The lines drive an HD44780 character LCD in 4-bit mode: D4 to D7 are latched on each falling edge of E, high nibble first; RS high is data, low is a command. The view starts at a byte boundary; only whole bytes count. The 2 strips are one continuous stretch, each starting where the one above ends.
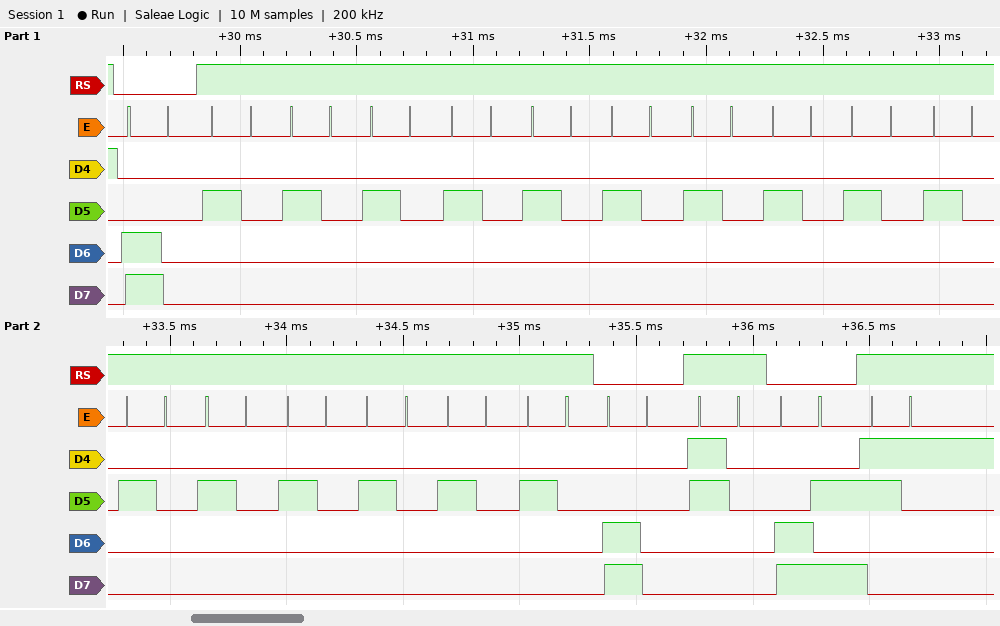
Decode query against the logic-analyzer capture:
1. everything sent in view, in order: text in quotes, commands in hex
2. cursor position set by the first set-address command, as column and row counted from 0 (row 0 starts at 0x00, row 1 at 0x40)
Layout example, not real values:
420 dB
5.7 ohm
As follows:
0xC0 "                " 0xC0 "0" 0xCA "1"
column 0, row 1
